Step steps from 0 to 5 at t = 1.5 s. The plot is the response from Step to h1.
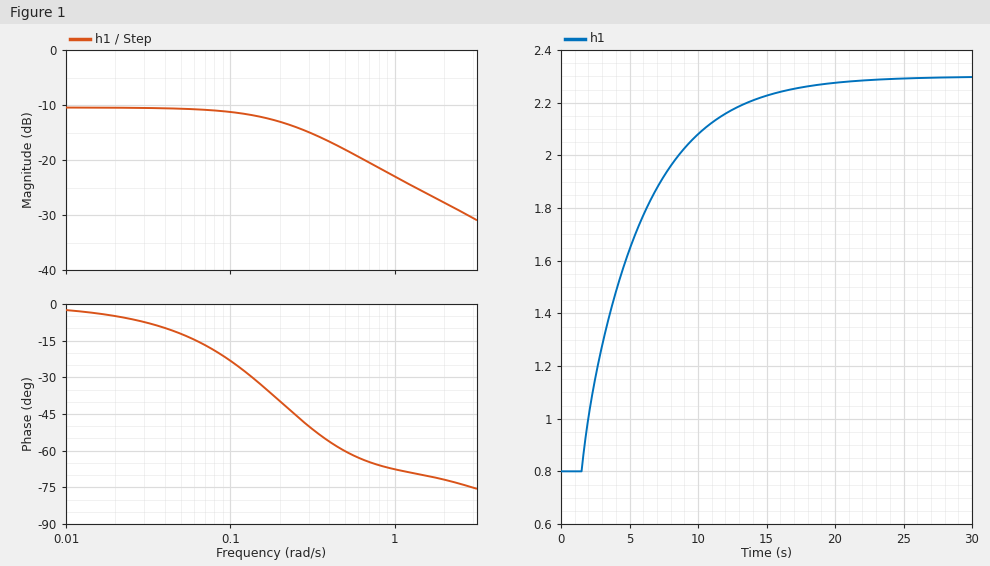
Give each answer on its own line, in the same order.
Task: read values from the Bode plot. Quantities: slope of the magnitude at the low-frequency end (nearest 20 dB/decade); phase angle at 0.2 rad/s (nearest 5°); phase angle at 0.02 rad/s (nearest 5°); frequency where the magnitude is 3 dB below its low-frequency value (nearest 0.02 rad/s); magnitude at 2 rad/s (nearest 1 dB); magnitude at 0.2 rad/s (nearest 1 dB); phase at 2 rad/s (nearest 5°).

0 dB/decade
-40°
-5°
0.22 rad/s
-28 dB
-13 dB
-70°
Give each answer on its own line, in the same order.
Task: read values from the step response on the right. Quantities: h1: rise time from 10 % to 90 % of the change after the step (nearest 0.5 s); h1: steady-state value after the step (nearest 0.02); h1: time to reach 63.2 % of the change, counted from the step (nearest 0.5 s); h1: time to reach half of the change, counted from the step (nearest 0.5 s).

10.0 s
2.30
4.5 s
3.0 s
